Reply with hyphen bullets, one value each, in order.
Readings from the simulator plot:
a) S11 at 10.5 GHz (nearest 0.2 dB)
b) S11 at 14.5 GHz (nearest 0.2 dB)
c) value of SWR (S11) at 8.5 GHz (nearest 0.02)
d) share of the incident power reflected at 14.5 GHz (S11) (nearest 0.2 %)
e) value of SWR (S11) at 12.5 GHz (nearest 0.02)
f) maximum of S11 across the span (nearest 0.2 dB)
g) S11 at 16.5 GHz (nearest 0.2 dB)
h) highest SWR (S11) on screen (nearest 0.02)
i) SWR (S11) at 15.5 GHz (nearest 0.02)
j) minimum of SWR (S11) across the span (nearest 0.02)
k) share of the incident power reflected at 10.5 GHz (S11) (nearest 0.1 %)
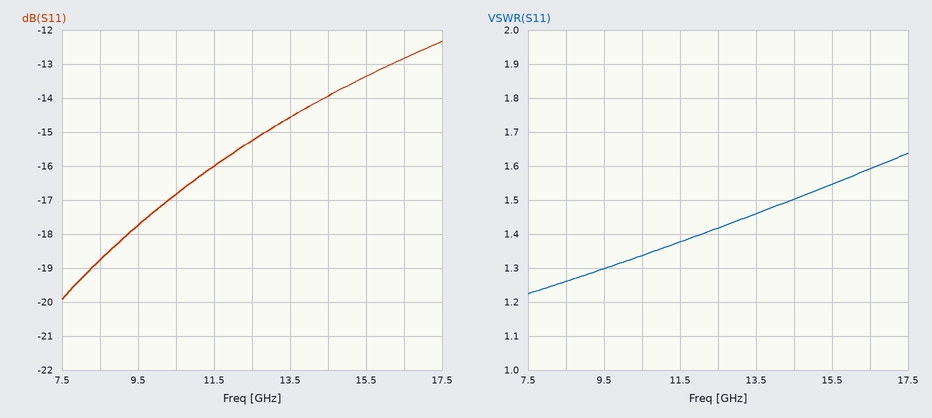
- -16.8 dB
- -14.0 dB
- 1.26
- 4.0 %
- 1.42
- -12.4 dB
- -12.8 dB
- 1.64
- 1.54
- 1.22
- 2.1 %
